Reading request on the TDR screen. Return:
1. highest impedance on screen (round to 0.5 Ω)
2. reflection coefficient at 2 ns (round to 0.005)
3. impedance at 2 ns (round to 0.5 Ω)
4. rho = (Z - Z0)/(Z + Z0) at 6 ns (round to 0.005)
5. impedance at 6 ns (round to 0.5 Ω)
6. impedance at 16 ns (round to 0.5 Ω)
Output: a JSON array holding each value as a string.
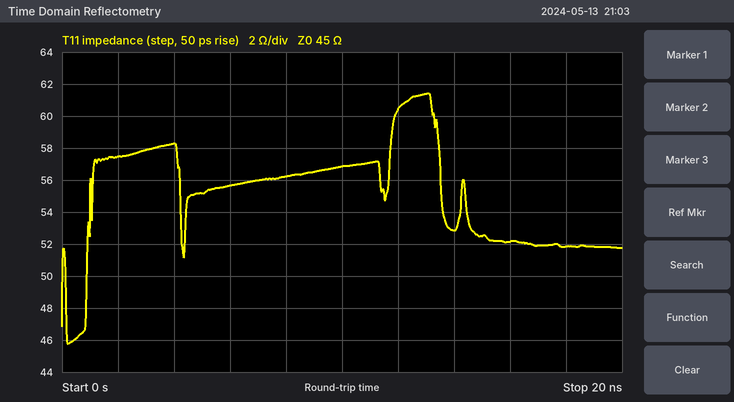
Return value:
["61.5 Ω", "+0.120", "57.5 Ω", "+0.105", "55.5 Ω", "52.0 Ω"]
